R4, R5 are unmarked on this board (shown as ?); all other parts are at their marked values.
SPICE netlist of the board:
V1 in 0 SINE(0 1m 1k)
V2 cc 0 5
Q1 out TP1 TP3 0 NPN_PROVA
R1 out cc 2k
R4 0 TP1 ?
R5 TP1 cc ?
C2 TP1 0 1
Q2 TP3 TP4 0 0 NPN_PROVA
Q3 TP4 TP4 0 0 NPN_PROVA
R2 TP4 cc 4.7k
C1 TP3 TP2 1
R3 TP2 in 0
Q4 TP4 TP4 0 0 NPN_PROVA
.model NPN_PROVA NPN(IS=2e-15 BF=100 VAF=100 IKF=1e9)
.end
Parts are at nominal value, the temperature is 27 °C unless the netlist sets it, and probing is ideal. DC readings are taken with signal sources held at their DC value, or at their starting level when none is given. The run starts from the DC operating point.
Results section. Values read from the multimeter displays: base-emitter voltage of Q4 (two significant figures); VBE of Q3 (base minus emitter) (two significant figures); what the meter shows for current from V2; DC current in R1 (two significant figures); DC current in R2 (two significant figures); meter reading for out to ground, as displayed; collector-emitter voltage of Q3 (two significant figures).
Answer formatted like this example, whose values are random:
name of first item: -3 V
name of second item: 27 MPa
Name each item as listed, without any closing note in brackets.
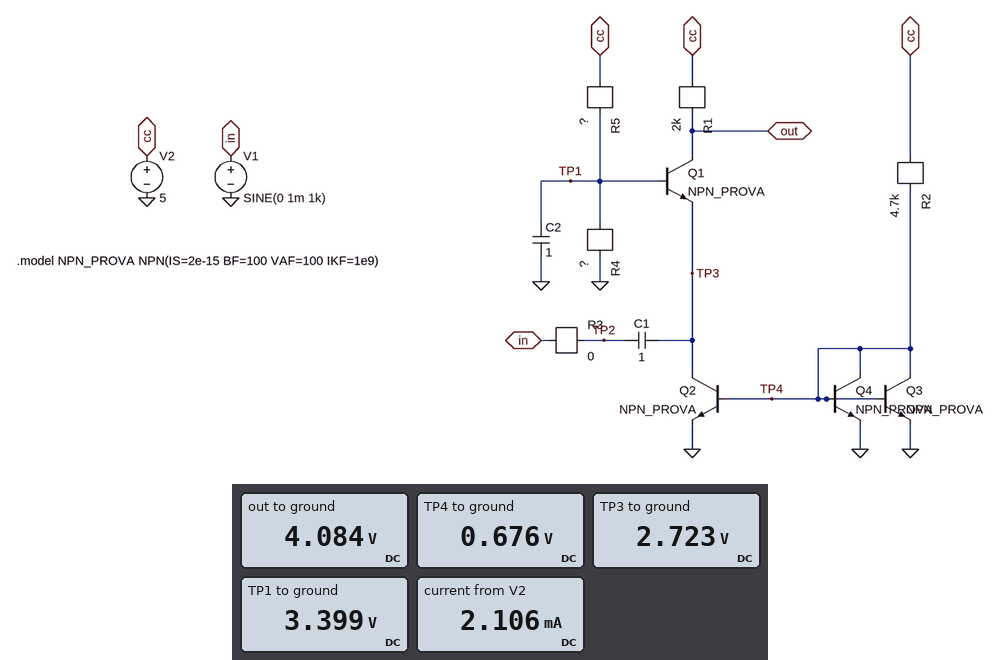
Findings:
base-emitter voltage of Q4: 680 mV
VBE of Q3 (base minus emitter): 680 mV
what the meter shows for current from V2: 2.106 mA
DC current in R1: 460 µA
DC current in R2: 920 µA
meter reading for out to ground, as displayed: 4.084 V
collector-emitter voltage of Q3: 680 mV
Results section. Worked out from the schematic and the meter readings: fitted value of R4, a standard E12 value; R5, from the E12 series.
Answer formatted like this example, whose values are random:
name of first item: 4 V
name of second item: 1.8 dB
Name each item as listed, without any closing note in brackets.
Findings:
fitted value of R4, a standard E12 value: 4.7 kΩ
R5, from the E12 series: 2.2 kΩ
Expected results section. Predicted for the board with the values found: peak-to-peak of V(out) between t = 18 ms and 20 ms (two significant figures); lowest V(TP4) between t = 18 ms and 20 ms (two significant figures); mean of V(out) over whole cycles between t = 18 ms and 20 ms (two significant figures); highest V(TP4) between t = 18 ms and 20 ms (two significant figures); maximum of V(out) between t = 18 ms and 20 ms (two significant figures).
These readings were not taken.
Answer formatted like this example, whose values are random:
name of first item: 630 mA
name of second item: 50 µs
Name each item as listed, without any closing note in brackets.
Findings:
peak-to-peak of V(out) between t = 18 ms and 20 ms: 70 mV
lowest V(TP4) between t = 18 ms and 20 ms: 680 mV
mean of V(out) over whole cycles between t = 18 ms and 20 ms: 4.1 V
highest V(TP4) between t = 18 ms and 20 ms: 680 mV
maximum of V(out) between t = 18 ms and 20 ms: 4.1 V
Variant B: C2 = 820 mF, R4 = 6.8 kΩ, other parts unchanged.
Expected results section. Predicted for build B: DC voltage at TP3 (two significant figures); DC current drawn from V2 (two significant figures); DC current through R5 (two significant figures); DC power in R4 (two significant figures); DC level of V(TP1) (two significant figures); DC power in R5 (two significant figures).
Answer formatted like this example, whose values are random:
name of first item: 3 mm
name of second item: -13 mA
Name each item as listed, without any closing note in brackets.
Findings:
DC voltage at TP3: 3.1 V
DC current drawn from V2: 1.9 mA
DC current through R5: 560 µA
DC power in R4: 2.1 mW
DC level of V(TP1): 3.8 V
DC power in R5: 690 µW
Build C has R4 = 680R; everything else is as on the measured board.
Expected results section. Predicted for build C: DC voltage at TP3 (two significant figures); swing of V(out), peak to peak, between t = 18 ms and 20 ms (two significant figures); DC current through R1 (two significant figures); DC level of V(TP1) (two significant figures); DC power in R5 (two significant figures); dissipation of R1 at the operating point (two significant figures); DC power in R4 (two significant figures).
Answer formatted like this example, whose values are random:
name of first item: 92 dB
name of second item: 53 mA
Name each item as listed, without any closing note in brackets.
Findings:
DC voltage at TP3: 500 mV
swing of V(out), peak to peak, between t = 18 ms and 20 ms: 69 mV
DC current through R1: 450 µA
DC level of V(TP1): 1.2 V
DC power in R5: 6.6 mW
dissipation of R1 at the operating point: 400 µW
DC power in R4: 2.0 mW
